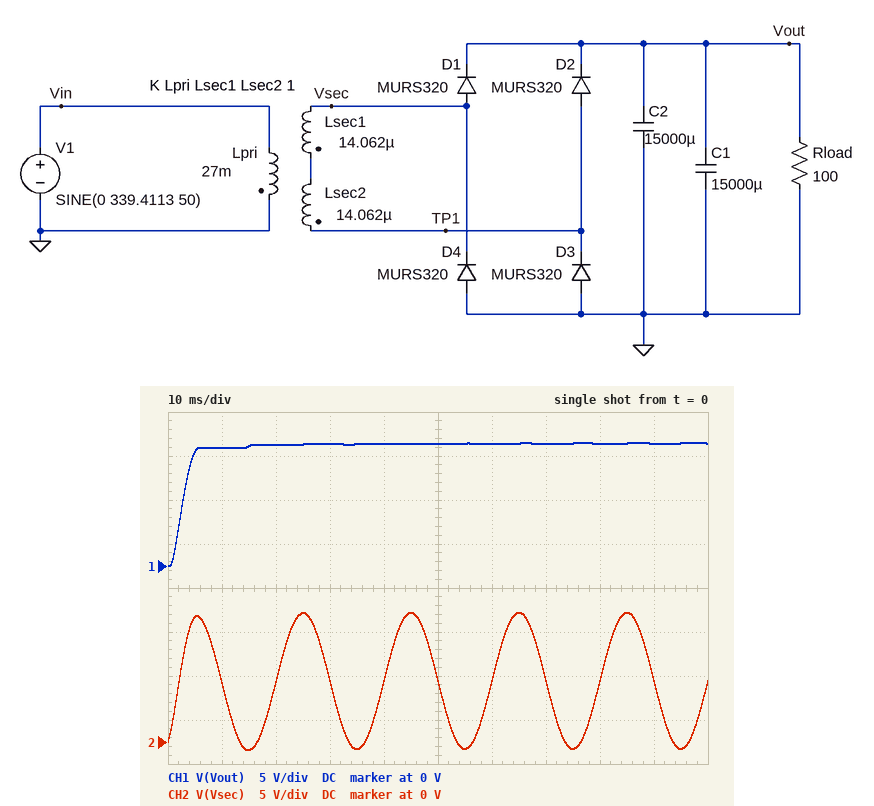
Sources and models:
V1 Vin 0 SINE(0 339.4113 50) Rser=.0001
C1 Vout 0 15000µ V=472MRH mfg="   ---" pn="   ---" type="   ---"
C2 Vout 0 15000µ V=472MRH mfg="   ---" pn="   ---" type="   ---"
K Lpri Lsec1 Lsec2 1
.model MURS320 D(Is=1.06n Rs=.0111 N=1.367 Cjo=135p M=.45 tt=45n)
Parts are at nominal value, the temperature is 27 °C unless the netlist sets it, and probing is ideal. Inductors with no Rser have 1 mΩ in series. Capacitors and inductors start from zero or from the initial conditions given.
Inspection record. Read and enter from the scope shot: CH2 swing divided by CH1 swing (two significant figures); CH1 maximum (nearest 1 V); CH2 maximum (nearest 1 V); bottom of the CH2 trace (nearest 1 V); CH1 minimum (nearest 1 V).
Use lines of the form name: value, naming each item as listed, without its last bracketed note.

CH2 swing divided by CH1 swing: 1.1
CH1 maximum: 14 V
CH2 maximum: 15 V
bottom of the CH2 trace: -1 V
CH1 minimum: 0 V
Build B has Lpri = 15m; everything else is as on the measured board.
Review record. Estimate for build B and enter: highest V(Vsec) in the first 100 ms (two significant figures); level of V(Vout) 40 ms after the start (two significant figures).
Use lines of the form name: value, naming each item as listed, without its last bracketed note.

highest V(Vsec) in the first 100 ms: 20 V
level of V(Vout) 40 ms after the start: 19 V
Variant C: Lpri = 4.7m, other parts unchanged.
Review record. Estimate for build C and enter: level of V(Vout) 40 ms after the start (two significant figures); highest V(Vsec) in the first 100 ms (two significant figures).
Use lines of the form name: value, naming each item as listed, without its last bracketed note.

level of V(Vout) 40 ms after the start: 35 V
highest V(Vsec) in the first 100 ms: 36 V
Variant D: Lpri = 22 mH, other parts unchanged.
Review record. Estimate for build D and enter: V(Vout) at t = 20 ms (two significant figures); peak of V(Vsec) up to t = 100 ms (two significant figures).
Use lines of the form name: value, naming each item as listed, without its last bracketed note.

V(Vout) at t = 20 ms: 15 V
peak of V(Vsec) up to t = 100 ms: 16 V
